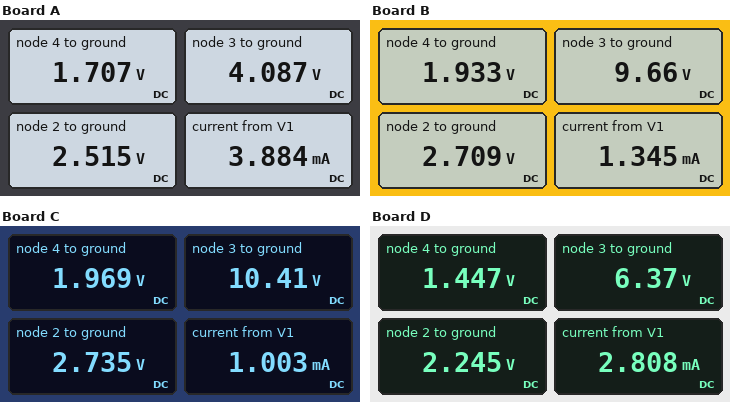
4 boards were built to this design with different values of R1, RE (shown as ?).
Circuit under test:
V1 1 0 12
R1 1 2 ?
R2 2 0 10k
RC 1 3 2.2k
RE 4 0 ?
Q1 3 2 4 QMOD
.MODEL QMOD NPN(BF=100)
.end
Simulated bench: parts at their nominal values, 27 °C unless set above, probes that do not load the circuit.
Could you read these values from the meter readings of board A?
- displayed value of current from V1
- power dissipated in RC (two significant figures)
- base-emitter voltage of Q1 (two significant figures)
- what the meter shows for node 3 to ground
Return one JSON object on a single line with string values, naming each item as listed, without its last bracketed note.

{"displayed value of current from V1": "3.884 mA", "power dissipated in RC": "28 mW", "base-emitter voltage of Q1": "810 mV", "what the meter shows for node 3 to ground": "4.087 V"}
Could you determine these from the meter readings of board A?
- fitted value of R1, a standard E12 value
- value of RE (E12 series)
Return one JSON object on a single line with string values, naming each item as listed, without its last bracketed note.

{"fitted value of R1, a standard E12 value": "33 kΩ", "value of RE": "470 Ω"}
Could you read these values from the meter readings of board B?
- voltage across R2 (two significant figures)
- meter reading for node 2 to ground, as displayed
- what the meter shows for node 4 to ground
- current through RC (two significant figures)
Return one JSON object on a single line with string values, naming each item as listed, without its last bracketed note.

{"voltage across R2": "2.7 V", "meter reading for node 2 to ground, as displayed": "2.709 V", "what the meter shows for node 4 to ground": "1.933 V", "current through RC": "1.1 mA"}
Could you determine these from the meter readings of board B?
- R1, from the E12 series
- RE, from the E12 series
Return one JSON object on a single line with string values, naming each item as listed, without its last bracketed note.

{"R1, from the E12 series": "33 kΩ", "RE, from the E12 series": "1.8 kΩ"}
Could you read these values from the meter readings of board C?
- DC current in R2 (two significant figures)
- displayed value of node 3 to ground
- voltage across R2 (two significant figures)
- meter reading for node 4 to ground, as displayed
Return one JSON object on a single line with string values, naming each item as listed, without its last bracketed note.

{"DC current in R2": "270 µA", "displayed value of node 3 to ground": "10.41 V", "voltage across R2": "2.7 V", "meter reading for node 4 to ground, as displayed": "1.969 V"}
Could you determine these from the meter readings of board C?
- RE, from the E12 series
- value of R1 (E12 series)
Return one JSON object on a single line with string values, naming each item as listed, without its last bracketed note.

{"RE, from the E12 series": "2.7 kΩ", "value of R1": "33 kΩ"}
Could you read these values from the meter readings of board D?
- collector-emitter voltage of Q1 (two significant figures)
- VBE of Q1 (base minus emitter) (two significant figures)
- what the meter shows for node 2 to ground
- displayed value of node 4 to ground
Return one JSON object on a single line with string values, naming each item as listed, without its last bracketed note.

{"collector-emitter voltage of Q1": "4.9 V", "VBE of Q1 (base minus emitter)": "800 mV", "what the meter shows for node 2 to ground": "2.245 V", "displayed value of node 4 to ground": "1.447 V"}
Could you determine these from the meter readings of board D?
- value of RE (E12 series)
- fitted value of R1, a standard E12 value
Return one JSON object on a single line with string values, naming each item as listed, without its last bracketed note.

{"value of RE": "560 Ω", "fitted value of R1, a standard E12 value": "39 kΩ"}
